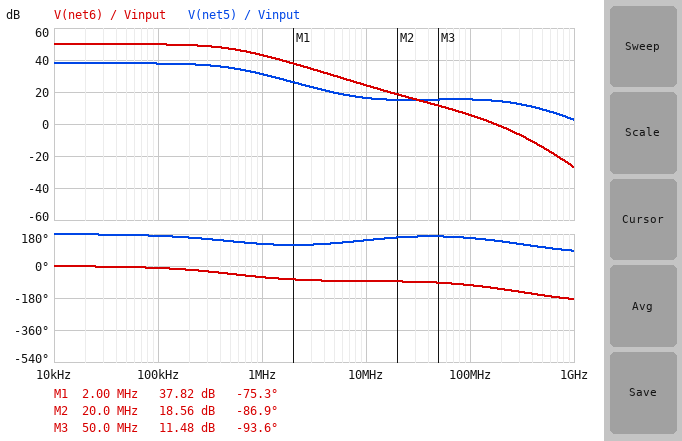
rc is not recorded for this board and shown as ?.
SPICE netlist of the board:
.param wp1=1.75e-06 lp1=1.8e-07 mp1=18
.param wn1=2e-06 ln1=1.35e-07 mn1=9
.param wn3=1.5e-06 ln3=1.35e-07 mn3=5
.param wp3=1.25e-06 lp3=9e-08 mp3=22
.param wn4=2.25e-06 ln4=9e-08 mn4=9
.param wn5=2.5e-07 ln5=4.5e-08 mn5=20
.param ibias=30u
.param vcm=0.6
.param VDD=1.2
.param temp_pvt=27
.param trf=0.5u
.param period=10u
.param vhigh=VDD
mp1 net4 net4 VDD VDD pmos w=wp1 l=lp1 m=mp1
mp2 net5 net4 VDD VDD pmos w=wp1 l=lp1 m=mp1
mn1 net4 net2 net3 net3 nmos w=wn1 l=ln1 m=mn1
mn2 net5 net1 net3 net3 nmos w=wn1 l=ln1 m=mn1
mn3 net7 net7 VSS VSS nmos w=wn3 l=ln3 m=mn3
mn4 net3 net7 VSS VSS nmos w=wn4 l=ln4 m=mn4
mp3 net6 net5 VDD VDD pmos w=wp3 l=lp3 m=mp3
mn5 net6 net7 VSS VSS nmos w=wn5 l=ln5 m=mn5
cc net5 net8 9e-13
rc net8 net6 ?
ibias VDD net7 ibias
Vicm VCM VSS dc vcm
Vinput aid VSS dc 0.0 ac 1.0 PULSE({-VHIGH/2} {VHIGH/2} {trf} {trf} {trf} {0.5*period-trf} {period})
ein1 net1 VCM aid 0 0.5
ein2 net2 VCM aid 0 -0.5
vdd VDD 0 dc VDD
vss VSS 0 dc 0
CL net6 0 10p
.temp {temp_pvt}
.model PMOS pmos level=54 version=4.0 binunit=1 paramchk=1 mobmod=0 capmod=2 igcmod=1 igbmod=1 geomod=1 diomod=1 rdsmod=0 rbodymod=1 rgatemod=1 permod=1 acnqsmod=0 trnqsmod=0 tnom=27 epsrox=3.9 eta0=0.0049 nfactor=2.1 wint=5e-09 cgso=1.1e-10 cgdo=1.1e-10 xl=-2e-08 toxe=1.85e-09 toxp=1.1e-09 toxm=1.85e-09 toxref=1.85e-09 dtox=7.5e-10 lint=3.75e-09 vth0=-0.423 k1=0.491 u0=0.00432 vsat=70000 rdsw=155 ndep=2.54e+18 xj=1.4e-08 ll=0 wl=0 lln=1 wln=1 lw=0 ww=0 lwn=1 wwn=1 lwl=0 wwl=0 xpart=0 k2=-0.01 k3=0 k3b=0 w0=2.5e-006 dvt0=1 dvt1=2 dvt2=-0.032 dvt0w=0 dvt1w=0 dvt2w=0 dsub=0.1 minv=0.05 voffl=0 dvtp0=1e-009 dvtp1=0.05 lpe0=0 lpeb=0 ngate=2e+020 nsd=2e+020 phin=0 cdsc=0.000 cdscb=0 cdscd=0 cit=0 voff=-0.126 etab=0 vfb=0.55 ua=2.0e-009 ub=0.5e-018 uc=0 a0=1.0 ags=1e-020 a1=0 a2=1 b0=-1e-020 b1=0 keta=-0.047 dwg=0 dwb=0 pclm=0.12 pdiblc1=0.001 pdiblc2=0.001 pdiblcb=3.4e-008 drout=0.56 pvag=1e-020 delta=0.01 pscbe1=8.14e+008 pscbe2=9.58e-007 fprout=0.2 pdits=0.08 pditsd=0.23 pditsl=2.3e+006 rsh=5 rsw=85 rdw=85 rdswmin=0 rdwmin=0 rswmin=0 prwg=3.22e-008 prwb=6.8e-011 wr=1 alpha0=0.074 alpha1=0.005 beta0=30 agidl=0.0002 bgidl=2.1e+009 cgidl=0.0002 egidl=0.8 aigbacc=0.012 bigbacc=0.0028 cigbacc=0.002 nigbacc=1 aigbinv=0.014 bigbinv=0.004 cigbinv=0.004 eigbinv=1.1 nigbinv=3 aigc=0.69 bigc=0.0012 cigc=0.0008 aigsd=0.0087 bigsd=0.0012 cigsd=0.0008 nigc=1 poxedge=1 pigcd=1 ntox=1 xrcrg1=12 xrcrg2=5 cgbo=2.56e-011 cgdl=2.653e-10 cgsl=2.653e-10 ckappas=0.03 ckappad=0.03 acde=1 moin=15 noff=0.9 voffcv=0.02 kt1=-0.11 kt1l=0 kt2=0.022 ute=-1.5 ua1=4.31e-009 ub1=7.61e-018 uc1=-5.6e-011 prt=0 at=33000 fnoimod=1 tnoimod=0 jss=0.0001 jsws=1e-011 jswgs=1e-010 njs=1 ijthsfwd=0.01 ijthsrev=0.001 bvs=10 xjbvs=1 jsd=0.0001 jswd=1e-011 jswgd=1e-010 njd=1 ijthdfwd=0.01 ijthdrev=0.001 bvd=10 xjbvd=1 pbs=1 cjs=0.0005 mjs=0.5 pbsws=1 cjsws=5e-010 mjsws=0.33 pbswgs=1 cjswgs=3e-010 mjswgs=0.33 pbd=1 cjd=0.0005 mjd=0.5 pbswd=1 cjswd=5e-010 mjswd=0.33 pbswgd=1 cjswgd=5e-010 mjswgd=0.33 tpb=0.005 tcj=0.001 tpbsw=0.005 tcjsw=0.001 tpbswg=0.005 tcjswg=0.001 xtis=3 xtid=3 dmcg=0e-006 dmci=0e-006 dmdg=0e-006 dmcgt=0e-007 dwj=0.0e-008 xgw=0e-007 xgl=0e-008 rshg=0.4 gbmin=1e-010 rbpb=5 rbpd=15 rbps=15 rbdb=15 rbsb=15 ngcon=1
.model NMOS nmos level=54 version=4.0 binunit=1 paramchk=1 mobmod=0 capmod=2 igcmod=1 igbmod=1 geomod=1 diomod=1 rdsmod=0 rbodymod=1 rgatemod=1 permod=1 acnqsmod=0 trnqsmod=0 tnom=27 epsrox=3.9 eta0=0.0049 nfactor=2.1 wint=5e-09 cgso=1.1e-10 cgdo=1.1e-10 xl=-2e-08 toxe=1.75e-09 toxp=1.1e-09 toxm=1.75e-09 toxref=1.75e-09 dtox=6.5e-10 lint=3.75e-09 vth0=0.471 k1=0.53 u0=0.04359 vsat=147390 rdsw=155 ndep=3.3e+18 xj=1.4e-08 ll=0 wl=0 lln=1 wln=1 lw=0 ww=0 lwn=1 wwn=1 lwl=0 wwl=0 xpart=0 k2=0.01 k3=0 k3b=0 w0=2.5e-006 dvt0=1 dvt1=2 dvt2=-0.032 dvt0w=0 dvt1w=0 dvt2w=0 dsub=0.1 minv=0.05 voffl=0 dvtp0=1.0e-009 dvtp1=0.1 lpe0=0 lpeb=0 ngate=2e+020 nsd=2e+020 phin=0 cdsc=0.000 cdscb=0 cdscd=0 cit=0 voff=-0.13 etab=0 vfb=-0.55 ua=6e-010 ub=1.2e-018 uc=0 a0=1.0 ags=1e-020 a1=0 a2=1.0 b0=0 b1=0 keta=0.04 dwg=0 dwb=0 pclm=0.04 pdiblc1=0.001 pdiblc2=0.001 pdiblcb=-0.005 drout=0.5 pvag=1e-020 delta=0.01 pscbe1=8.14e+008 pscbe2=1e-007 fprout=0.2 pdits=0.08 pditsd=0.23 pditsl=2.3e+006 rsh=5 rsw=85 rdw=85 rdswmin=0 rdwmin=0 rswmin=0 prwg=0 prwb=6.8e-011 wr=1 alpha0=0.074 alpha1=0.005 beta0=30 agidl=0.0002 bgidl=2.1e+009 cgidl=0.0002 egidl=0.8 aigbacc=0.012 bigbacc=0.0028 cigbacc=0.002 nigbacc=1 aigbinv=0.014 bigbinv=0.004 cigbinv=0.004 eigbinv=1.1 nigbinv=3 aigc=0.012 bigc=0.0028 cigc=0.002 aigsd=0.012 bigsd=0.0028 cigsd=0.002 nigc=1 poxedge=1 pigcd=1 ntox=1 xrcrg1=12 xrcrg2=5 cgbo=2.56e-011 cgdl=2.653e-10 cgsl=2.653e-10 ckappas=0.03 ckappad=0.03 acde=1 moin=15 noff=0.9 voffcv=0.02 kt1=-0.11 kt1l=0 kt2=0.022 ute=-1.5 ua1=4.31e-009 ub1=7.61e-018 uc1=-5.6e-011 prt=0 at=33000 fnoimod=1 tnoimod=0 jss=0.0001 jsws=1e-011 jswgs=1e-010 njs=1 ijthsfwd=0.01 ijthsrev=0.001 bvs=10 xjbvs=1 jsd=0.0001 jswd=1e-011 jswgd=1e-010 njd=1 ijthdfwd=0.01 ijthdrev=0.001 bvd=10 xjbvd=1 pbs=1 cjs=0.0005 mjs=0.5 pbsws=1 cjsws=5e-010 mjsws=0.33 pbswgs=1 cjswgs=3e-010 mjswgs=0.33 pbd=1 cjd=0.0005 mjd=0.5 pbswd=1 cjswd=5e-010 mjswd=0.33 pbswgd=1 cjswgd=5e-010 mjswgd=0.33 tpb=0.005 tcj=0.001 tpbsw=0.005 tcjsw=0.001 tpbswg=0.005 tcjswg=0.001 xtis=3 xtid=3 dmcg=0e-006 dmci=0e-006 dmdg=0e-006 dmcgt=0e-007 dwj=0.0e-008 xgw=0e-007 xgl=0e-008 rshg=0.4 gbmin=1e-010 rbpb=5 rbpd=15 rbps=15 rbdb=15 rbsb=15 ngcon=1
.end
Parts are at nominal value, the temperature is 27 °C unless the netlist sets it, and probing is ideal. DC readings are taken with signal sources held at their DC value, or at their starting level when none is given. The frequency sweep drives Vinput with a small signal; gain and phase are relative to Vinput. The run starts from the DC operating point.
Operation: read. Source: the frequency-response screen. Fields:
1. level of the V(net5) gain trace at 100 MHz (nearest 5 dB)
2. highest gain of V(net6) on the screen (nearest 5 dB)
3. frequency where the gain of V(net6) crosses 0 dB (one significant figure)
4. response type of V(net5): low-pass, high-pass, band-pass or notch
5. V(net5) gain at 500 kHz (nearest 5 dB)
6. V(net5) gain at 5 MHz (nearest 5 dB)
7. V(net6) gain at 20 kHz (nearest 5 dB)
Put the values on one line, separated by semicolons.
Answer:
15 dB; 50 dB; 200 MHz; low-pass; 35 dB; 20 dB; 50 dB
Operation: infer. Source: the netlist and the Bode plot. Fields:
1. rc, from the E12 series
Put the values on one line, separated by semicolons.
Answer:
5.6 kΩ
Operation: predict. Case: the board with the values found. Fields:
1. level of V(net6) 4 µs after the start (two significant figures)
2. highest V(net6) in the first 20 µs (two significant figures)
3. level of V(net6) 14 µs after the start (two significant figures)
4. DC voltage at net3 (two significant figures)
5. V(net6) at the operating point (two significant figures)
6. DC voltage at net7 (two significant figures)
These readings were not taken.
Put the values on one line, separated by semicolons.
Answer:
1.1 V; 1.1 V; 1.1 V; 170 mV; 210 mV; 430 mV
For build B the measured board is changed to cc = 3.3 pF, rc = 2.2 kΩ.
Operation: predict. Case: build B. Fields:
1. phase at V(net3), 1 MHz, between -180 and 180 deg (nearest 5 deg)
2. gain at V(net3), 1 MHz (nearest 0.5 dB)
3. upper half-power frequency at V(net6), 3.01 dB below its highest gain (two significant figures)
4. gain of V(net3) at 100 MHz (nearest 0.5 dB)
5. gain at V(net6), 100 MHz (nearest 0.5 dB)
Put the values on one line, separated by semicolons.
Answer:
105 deg; -27.0 dB; 150 kHz; -40.5 dB; -3.0 dB
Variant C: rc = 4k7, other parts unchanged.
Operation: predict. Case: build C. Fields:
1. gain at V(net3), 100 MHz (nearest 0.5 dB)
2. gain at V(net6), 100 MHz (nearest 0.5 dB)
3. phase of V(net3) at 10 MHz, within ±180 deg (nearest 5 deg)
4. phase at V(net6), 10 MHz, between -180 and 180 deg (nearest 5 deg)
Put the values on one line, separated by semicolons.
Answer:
-33.0 dB; 4.5 dB; 145 deg; -90 deg
